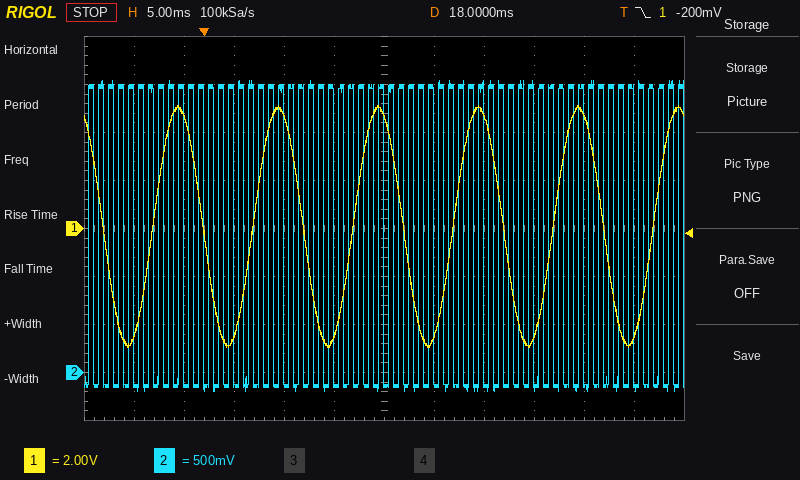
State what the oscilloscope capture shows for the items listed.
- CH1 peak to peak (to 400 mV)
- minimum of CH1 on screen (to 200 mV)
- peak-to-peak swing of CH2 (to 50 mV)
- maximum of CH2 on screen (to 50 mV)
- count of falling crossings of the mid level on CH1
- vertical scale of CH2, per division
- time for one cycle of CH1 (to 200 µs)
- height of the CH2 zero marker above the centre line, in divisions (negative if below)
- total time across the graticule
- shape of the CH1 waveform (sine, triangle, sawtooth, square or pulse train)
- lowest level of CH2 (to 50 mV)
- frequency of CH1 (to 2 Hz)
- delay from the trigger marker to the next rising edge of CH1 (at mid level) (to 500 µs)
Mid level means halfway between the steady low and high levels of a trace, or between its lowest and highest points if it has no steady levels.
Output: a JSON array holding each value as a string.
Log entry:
["10.0 V", "-5.0 V", "3.25 V", "3.05 V", "6", "500 mV", "10.0 ms", "-3.0 div", "60 ms", "sine", "-200 mV", "100 Hz", "5.0 ms"]
